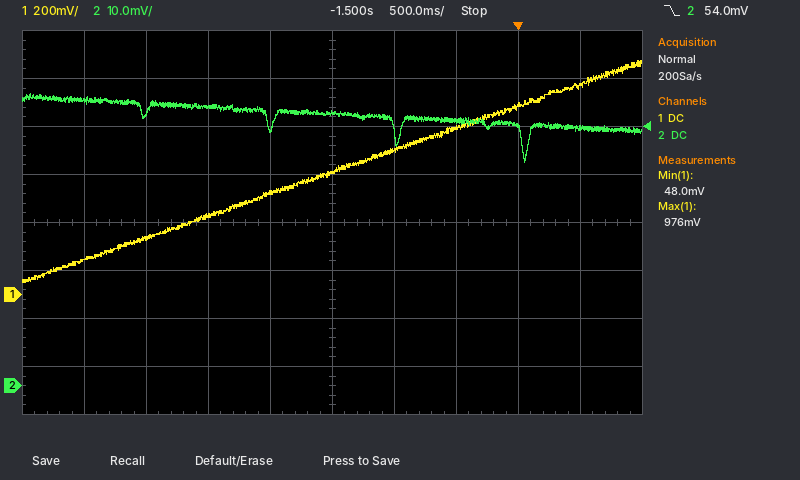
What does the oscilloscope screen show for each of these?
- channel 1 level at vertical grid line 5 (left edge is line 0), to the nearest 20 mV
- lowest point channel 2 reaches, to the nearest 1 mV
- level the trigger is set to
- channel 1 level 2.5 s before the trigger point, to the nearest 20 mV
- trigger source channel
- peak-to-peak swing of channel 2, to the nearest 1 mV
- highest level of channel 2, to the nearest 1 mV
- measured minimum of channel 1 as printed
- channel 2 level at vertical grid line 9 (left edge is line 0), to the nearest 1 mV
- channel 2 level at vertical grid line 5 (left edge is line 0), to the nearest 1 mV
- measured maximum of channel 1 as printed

500 mV
47 mV
54.0 mV
320 mV
channel 2
14 mV
61 mV
48.0 mV
54 mV
57 mV
976 mV
